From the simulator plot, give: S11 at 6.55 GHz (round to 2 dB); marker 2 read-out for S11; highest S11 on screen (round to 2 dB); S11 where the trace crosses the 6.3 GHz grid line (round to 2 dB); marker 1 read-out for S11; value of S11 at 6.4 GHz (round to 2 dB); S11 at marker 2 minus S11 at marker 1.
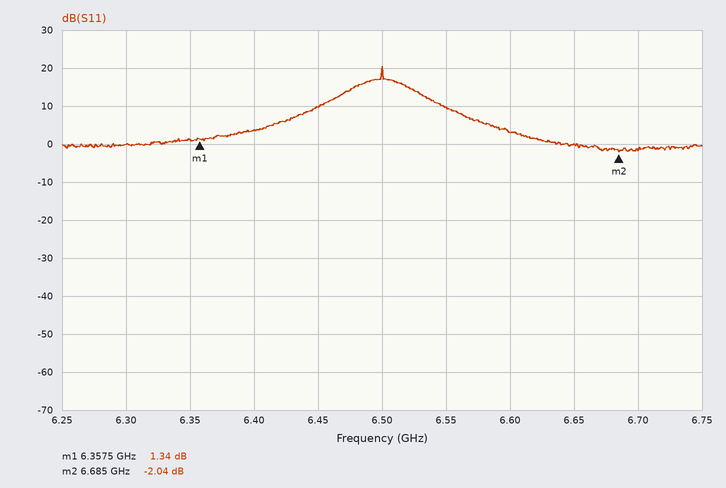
10 dB
-2.04 dB
20 dB
0 dB
1.34 dB
4 dB
-3.38 dB
